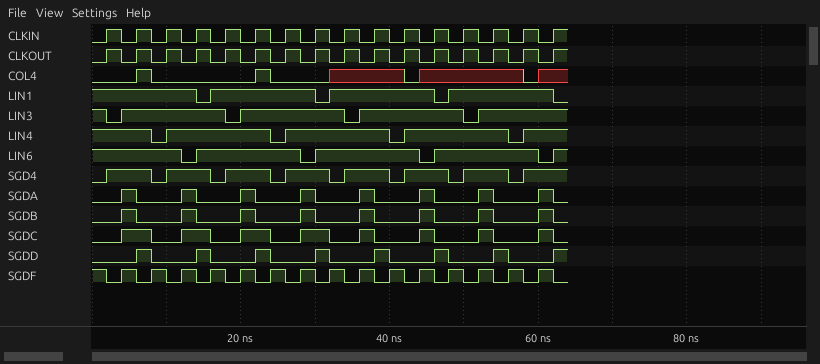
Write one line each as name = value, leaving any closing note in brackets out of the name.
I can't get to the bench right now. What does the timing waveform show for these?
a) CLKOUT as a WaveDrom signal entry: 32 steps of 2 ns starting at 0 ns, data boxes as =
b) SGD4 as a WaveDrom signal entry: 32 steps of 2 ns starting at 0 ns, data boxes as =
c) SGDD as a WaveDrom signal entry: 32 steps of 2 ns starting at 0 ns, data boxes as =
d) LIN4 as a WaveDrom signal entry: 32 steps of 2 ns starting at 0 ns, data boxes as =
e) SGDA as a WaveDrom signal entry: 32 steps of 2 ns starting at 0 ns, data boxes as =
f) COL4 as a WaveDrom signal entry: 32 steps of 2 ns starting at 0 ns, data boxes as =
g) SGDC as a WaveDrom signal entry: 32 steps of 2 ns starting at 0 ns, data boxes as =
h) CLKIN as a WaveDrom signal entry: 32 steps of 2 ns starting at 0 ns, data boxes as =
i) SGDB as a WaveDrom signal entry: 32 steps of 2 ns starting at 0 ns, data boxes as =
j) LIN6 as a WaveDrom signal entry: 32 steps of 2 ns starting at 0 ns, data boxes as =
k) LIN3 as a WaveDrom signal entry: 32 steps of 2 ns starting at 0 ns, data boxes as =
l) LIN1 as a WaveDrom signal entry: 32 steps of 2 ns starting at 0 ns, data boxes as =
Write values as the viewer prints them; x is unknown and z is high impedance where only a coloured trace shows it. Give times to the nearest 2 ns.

CLKOUT as a WaveDrom signal entry: 32 steps of 2 ns starting at 0 ns, data boxes as = = {name: 'CLKOUT', wave: '01010101010101010101010101010101'}
SGD4 as a WaveDrom signal entry: 32 steps of 2 ns starting at 0 ns, data boxes as = = {name: 'SGD4', wave: '01..01..01..01..01..01..01..01..'}
SGDD as a WaveDrom signal entry: 32 steps of 2 ns starting at 0 ns, data boxes as = = {name: 'SGDD', wave: '0..10..10..10..10..10..10..10..1'}
LIN4 as a WaveDrom signal entry: 32 steps of 2 ns starting at 0 ns, data boxes as = = {name: 'LIN4', wave: '1...01......01......01......01..'}
SGDA as a WaveDrom signal entry: 32 steps of 2 ns starting at 0 ns, data boxes as = = {name: 'SGDA', wave: '0.10..10..10..10..10..10..10..10'}
COL4 as a WaveDrom signal entry: 32 steps of 2 ns starting at 0 ns, data boxes as = = {name: 'COL4', wave: '0..10......10...x....0x......0x.'}
SGDC as a WaveDrom signal entry: 32 steps of 2 ns starting at 0 ns, data boxes as = = {name: 'SGDC', wave: '0.1.0.1.0.1.0.1.0.10..10..10..10'}
CLKIN as a WaveDrom signal entry: 32 steps of 2 ns starting at 0 ns, data boxes as = = {name: 'CLKIN', wave: '01010101010101010101010101010101'}
SGDB as a WaveDrom signal entry: 32 steps of 2 ns starting at 0 ns, data boxes as = = {name: 'SGDB', wave: '0.10..10..10..10..10..10..10..10'}
LIN6 as a WaveDrom signal entry: 32 steps of 2 ns starting at 0 ns, data boxes as = = {name: 'LIN6', wave: '1.....01......01......01......01'}
LIN3 as a WaveDrom signal entry: 32 steps of 2 ns starting at 0 ns, data boxes as = = {name: 'LIN3', wave: '101......01......01......01.....'}
LIN1 as a WaveDrom signal entry: 32 steps of 2 ns starting at 0 ns, data boxes as = = {name: 'LIN1', wave: '1......01......01......01......0'}
